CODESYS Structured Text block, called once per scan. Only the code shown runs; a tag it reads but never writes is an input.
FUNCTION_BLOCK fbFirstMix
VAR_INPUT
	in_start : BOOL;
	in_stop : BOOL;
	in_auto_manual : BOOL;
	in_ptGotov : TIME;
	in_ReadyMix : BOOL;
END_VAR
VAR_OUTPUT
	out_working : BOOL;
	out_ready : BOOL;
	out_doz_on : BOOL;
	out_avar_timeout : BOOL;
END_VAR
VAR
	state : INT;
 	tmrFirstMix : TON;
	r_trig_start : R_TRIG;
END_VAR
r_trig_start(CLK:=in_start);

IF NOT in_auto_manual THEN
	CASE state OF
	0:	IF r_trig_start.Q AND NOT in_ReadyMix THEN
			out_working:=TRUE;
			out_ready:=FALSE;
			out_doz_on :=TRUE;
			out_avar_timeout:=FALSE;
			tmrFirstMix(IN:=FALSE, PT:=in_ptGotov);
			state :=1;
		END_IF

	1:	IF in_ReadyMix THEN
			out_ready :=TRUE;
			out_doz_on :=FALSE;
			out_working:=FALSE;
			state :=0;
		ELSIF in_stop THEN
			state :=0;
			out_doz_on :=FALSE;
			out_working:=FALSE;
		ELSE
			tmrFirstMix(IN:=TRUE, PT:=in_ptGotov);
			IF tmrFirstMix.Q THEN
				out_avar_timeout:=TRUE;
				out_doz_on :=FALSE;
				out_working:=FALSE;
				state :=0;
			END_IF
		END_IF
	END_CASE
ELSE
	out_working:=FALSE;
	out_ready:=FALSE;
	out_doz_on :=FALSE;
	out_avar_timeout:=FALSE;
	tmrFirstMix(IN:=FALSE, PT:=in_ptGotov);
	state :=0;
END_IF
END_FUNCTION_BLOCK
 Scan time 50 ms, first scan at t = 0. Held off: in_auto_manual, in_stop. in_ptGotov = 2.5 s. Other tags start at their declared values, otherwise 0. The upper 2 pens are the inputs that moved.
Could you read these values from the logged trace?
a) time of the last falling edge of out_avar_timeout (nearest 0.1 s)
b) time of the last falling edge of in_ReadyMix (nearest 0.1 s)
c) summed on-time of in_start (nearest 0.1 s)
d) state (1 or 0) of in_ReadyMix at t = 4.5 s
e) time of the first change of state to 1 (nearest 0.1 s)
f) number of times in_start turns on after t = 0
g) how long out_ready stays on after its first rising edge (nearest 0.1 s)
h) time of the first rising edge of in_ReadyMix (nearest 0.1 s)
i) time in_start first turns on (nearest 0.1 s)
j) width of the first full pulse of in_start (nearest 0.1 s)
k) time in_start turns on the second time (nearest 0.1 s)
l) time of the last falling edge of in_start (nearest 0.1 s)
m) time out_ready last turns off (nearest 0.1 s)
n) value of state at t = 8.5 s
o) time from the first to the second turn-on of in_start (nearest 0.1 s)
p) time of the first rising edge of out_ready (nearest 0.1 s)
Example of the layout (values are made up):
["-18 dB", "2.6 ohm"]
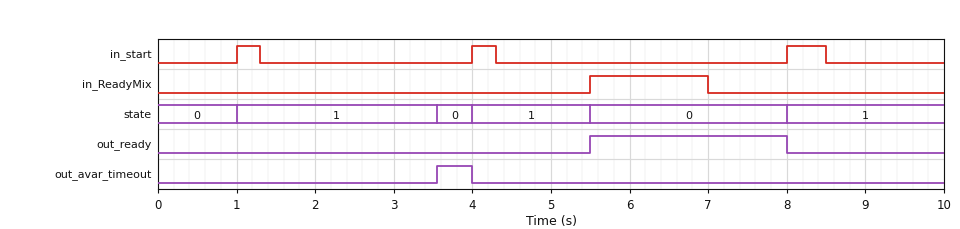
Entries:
["4.0 s", "7.0 s", "1.1 s", "0", "1.0 s", "3", "2.5 s", "5.5 s", "1.0 s", "0.3 s", "4.0 s", "8.5 s", "8.0 s", "1", "3.0 s", "5.5 s"]
